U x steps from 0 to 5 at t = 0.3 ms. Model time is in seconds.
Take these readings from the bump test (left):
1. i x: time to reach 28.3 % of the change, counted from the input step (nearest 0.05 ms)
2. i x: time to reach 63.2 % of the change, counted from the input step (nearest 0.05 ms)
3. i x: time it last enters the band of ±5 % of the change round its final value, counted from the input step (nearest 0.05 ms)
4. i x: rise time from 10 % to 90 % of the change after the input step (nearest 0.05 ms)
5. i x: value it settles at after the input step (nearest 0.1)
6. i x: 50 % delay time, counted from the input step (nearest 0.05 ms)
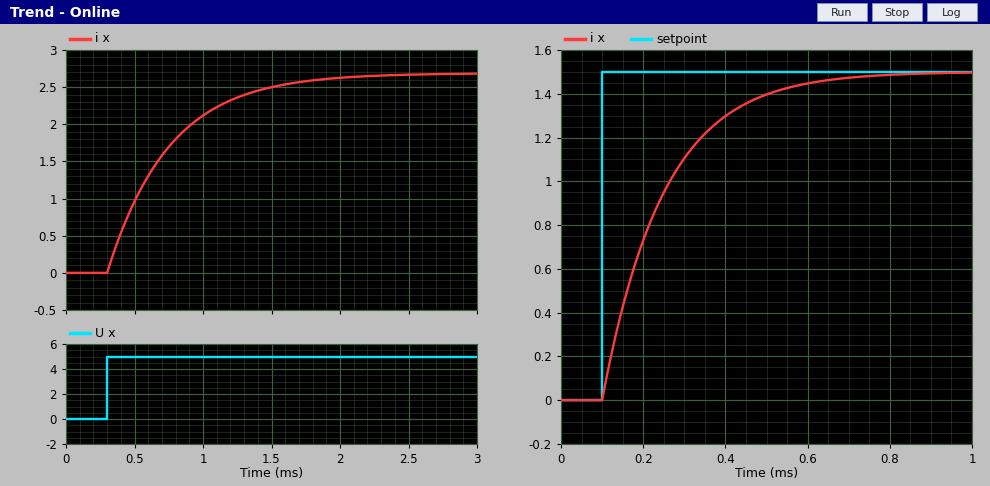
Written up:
0.15 ms
0.45 ms
1.35 ms
1.00 ms
2.7
0.30 ms
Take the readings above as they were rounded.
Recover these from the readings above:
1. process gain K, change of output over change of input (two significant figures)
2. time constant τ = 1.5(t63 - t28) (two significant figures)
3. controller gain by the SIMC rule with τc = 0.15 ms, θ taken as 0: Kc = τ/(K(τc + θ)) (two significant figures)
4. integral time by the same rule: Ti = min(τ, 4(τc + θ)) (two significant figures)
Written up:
0.54
0.45 ms
5.6
0.45 ms
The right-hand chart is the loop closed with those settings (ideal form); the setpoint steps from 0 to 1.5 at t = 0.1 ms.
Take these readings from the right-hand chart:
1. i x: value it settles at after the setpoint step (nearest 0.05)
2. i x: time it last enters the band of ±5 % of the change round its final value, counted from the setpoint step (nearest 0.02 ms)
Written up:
1.50
0.44 ms
